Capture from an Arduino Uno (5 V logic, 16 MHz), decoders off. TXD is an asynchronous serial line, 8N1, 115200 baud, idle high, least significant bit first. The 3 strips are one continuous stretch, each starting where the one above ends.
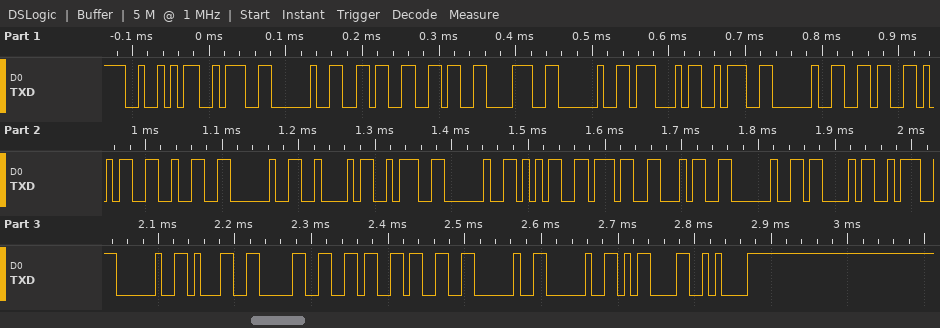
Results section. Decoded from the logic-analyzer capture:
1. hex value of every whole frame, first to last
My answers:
0x52 0x3A 0x20 0x36 0x36 0x38 0x20 0x47 0x3A 0x20 0x36 0x35 0x32 0x20 0x42 0x3A 0x20 0x35 0x37 0x34 0x20 0x43 0x3A 0x20 0x31 0x30 0x36 0x33 0x20 0x20 0x0D 0x0A
